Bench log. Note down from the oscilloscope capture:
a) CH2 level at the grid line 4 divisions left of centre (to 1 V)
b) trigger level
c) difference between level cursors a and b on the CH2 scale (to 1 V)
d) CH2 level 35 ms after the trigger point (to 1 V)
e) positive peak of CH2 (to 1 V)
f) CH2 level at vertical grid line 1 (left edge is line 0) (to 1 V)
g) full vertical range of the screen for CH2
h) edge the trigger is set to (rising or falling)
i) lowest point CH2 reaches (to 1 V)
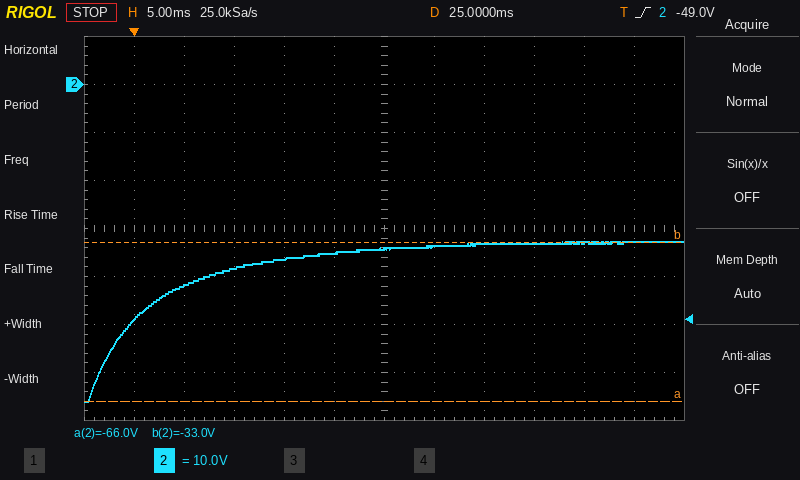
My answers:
-42 V
-49.0 V
33 V
-33 V
-33 V
-49 V
80 V
rising
-66 V
